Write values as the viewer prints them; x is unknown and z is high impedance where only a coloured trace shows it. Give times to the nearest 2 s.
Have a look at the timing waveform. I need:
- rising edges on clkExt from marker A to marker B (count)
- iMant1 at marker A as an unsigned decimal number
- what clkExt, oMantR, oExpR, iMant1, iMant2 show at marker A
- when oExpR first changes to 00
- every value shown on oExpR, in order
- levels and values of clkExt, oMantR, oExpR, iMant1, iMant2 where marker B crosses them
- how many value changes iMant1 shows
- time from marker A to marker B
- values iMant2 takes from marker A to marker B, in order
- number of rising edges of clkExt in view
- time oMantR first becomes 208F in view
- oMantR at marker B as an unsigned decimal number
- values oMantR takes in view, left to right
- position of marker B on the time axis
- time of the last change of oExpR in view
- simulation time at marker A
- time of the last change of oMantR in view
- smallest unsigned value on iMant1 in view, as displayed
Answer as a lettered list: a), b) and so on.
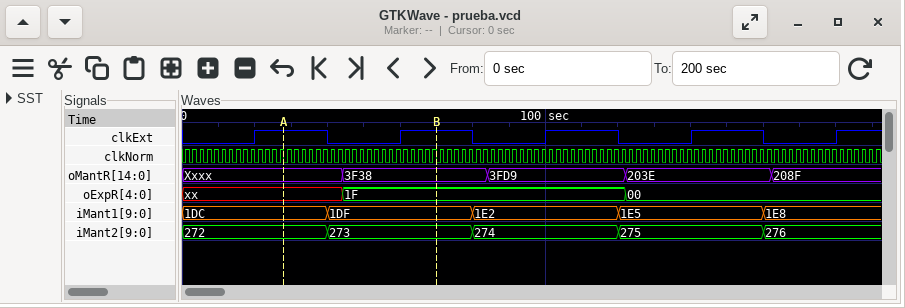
a) 1
b) 476
c) clkExt=1, oMantR=Xxxx, oExpR=xx, iMant1=1DC, iMant2=272
d) 122 s
e) xx, 1F, 00
f) clkExt=1, oMantR=3F38, oExpR=1F, iMant1=1DF, iMant2=273
g) 4
h) 42 s
i) 272, 273
j) 5
k) 162 s
l) 16184
m) Xxxx, 3F38, 3FD9, 203E, 208F
n) 70 s
o) 122 s
p) 28 s
q) 162 s
r) 1DC
